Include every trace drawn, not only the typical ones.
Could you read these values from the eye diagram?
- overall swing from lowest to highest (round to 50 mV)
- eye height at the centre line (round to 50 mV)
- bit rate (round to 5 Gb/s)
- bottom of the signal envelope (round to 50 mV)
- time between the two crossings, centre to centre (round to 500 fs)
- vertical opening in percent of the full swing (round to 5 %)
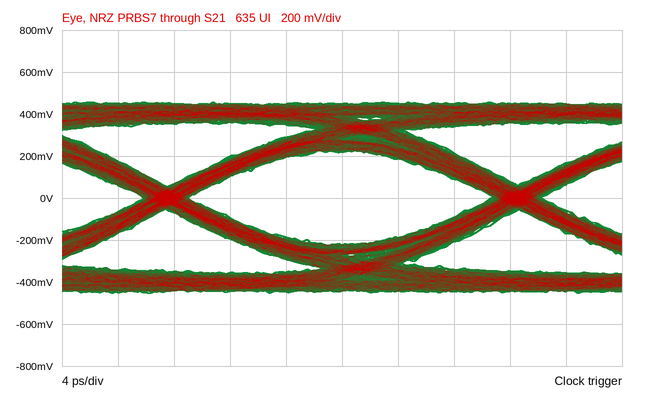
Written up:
900 mV
450 mV
40 Gb/s
-450 mV
25.0 ps
50 %
